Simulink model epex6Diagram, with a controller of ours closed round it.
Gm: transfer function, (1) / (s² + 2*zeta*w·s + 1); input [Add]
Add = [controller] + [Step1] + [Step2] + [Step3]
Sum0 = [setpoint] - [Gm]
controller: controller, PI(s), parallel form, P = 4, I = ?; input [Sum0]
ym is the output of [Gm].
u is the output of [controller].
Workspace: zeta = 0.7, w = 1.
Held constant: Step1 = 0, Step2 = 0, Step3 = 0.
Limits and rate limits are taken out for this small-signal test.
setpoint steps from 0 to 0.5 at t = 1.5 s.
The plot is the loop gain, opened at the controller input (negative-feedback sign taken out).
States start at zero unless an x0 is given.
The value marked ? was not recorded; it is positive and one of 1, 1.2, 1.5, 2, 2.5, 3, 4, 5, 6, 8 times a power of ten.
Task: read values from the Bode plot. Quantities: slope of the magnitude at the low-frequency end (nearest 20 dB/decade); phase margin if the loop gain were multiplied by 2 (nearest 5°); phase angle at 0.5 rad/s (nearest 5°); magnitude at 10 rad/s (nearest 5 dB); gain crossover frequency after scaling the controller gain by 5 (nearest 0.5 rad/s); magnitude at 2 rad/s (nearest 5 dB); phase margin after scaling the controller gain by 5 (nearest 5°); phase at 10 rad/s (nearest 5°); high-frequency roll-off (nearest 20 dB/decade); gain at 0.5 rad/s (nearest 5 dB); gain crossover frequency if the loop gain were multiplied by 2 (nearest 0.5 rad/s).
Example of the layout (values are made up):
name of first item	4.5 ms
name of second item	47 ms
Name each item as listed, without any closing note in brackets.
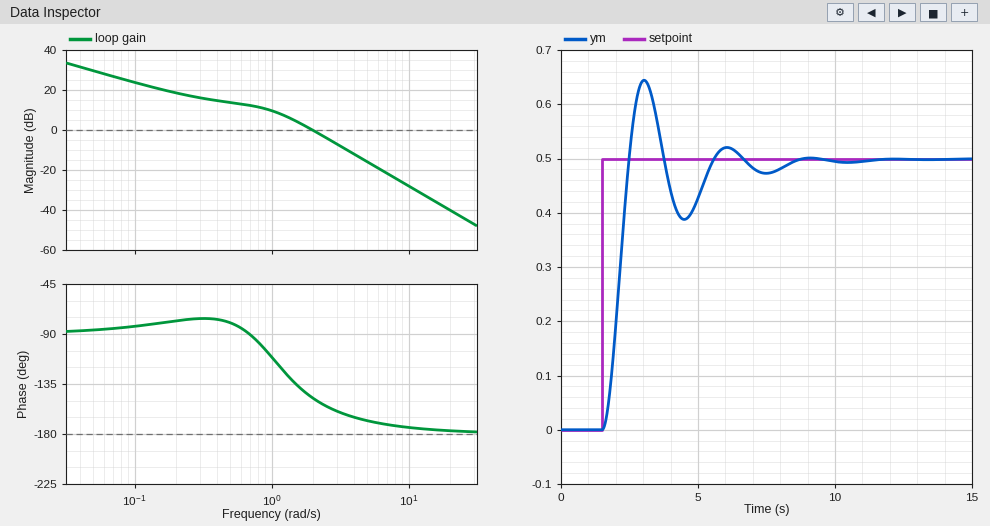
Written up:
slope of the magnitude at the low-frequency end	-20 dB/decade
phase margin if the loop gain were multiplied by 2	20°
phase angle at 0.5 rad/s	-80°
magnitude at 10 rad/s	-30 dB
gain crossover frequency after scaling the controller gain by 5	4.5 rad/s
magnitude at 2 rad/s	0 dB
phase margin after scaling the controller gain by 5	15°
phase at 10 rad/s	-175°
high-frequency roll-off	-40 dB/decade
gain at 0.5 rad/s	15 dB
gain crossover frequency if the loop gain were multiplied by 2	3.0 rad/s
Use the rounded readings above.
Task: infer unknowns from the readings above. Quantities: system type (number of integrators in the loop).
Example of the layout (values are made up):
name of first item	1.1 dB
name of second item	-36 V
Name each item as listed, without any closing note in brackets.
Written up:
system type	1
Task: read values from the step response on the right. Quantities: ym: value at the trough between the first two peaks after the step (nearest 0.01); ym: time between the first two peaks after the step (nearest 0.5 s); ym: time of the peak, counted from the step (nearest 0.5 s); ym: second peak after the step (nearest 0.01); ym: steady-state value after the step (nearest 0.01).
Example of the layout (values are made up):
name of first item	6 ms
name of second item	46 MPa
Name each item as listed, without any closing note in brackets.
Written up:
ym: value at the trough between the first two peaks after the step	0.39
ym: time between the first two peaks after the step	3.0 s
ym: time of the peak, counted from the step	1.5 s
ym: second peak after the step	0.52
ym: steady-state value after the step	0.50
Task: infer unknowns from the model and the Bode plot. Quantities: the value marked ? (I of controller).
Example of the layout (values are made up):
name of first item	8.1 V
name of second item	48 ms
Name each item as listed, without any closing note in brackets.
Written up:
the value marked ?	1.5
